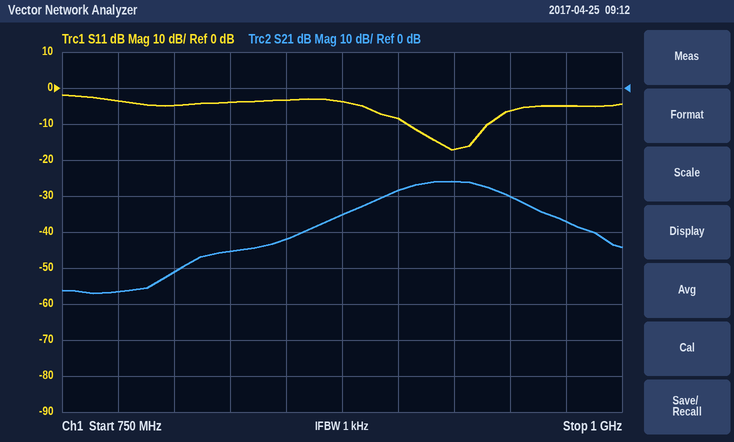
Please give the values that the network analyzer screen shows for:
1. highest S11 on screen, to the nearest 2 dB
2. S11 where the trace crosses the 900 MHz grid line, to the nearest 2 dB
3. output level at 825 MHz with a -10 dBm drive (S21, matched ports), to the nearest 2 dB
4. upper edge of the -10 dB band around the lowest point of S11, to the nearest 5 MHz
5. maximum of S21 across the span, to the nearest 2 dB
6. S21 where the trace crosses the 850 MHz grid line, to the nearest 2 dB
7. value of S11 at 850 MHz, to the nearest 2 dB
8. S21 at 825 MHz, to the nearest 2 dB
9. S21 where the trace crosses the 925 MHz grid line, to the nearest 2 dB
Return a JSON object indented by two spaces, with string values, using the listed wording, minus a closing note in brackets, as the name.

{
  "highest S11 on screen, to the nearest 2 dB": "-2 dB",
  "S11 where the trace crosses the 900 MHz grid line, to the nearest 2 dB": "-8 dB",
  "output level at 825 MHz with a -10 dBm drive (S21, matched ports), to the nearest 2 dB": "-56 dBm",
  "upper edge of the -10 dB band around the lowest point of S11, to the nearest 5 MHz": "940 MHz",
  "maximum of S21 across the span, to the nearest 2 dB": "-26 dB",
  "S21 where the trace crosses the 850 MHz grid line, to the nearest 2 dB": "-42 dB",
  "value of S11 at 850 MHz, to the nearest 2 dB": "-4 dB",
  "S21 at 825 MHz, to the nearest 2 dB": "-46 dB",
  "S21 where the trace crosses the 925 MHz grid line, to the nearest 2 dB": "-26 dB"
}
